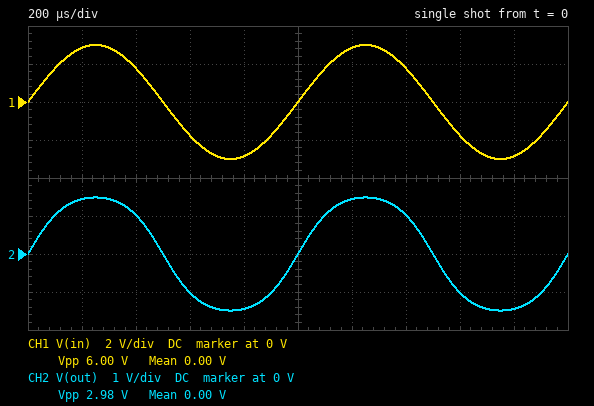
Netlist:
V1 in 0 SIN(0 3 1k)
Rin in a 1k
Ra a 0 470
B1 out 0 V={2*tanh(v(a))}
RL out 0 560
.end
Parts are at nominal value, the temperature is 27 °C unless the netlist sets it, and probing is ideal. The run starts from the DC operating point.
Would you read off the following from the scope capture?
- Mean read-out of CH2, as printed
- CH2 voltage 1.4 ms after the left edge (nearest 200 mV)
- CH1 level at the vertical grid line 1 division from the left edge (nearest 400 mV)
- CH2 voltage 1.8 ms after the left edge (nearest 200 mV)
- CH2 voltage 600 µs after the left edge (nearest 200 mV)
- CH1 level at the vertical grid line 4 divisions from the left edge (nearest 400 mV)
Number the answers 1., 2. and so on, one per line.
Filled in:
1. 0.00 V
2. 1.0 V
3. 2.8 V
4. -1.4 V
5. -1.0 V
6. -2.8 V
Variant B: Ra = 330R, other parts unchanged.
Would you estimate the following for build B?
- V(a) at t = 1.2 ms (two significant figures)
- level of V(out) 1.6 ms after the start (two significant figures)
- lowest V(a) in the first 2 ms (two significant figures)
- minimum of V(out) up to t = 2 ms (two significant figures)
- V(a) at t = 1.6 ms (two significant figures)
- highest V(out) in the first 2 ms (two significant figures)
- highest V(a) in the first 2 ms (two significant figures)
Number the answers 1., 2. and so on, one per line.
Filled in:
1. 710 mV
2. -820 mV
3. -740 mV
4. -1.3 V
5. -440 mV
6. 1.3 V
7. 740 mV
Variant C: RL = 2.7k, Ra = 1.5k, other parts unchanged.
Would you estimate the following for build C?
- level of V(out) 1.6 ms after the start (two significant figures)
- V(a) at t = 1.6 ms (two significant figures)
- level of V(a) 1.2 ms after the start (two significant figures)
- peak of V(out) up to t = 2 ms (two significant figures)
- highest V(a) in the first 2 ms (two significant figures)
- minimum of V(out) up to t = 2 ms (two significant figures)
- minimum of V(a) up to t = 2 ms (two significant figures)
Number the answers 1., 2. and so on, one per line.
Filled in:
1. -1.6 V
2. -1.1 V
3. 1.7 V
4. 1.9 V
5. 1.8 V
6. -1.9 V
7. -1.8 V
